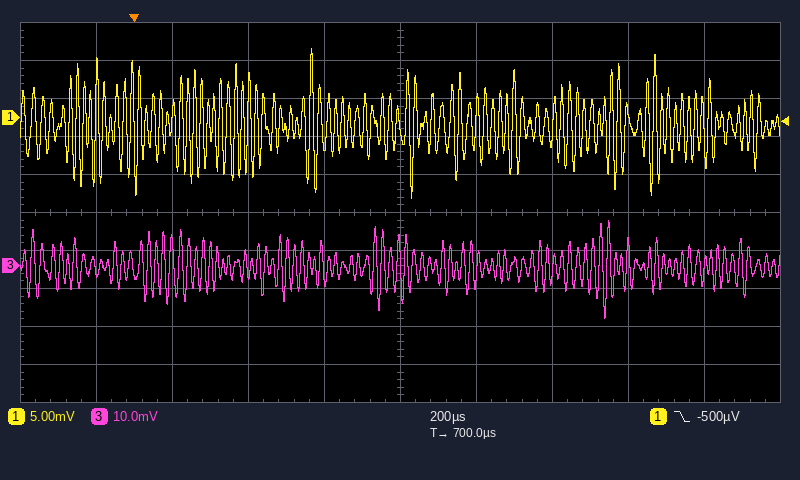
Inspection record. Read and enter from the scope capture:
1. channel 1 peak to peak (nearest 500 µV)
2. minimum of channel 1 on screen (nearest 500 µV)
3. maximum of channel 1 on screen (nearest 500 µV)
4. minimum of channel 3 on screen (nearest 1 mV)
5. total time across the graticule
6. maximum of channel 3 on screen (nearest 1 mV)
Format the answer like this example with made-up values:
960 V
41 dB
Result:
19.5 mV
-10.5 mV
9.0 mV
-14 mV
2 ms
12 mV
